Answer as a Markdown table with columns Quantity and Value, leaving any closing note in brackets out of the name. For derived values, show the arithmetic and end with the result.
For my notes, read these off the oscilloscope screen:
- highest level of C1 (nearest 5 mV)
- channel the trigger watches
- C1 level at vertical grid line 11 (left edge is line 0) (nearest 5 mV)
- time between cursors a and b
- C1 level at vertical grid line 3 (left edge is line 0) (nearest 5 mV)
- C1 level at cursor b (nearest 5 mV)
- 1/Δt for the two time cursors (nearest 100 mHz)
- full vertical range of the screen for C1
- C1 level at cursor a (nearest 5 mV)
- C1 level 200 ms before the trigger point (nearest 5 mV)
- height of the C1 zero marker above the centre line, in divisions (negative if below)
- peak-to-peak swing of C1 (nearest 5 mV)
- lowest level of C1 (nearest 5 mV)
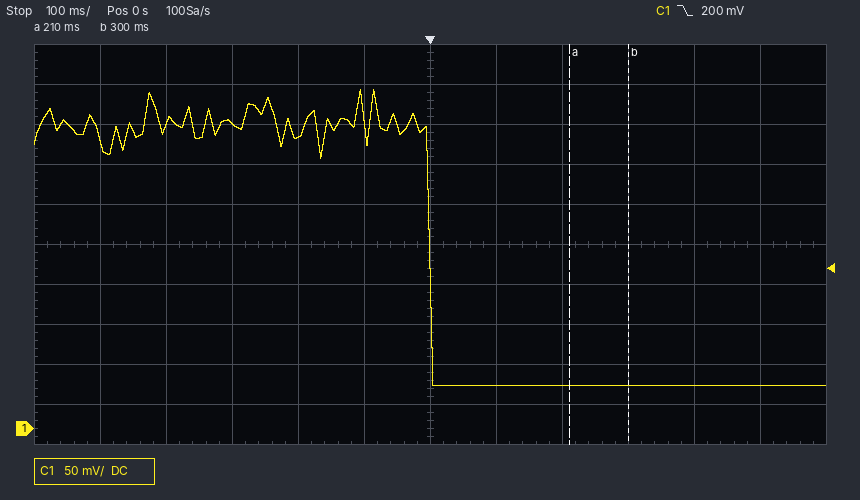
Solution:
| Quantity | Value |
|---|---|
| highest level of C1 | 425 mV |
| channel the trigger watches | C1 |
| C1 level at vertical grid line 11 (left edge is line 0) | 55 mV |
| time between cursors a and b | 300 ms − (210 ms) = 90 ms |
| C1 level at vertical grid line 3 (left edge is line 0) | 380 mV |
| C1 level at cursor b | 55 mV |
| 1/Δt for the two time cursors | 1 / 90 ms ≈ 11.1 Hz |
| full vertical range of the screen for C1 | 500 mV |
| C1 level at cursor a | 55 mV |
| C1 level 200 ms before the trigger point | 365 mV |
| height of the C1 zero marker above the centre line, in divisions | -4.6 div |
| peak-to-peak swing of C1 | 425 mV − (55 mV) = 370 mV |
| lowest level of C1 | 55 mV |
